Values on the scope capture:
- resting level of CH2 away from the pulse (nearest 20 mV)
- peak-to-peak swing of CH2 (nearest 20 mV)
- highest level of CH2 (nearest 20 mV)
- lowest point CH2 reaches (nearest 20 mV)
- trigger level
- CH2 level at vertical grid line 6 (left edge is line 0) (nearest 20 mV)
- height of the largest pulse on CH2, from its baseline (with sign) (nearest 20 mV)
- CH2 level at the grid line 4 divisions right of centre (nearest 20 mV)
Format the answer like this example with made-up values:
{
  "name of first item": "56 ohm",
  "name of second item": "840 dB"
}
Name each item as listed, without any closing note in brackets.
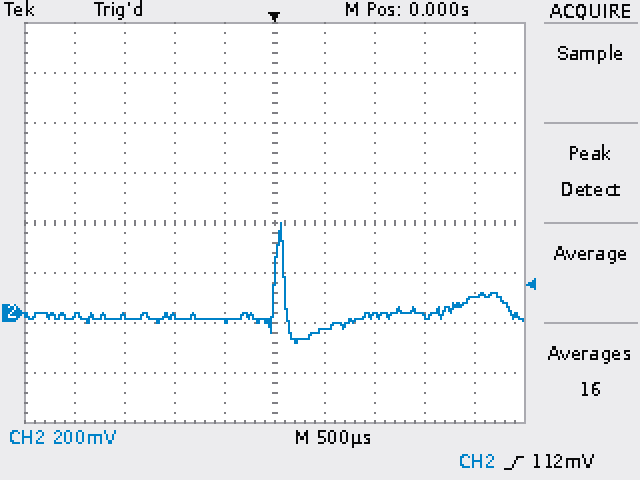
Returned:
{
  "resting level of CH2 away from the pulse": "-20 mV",
  "peak-to-peak swing of CH2": "480 mV",
  "highest level of CH2": "360 mV",
  "lowest point CH2 reaches": "-120 mV",
  "trigger level": "112 mV",
  "CH2 level at vertical grid line 6 (left edge is line 0)": "-60 mV",
  "height of the largest pulse on CH2, from its baseline (with sign)": "+380 mV",
  "CH2 level at the grid line 4 divisions right of centre": "60 mV"
}
